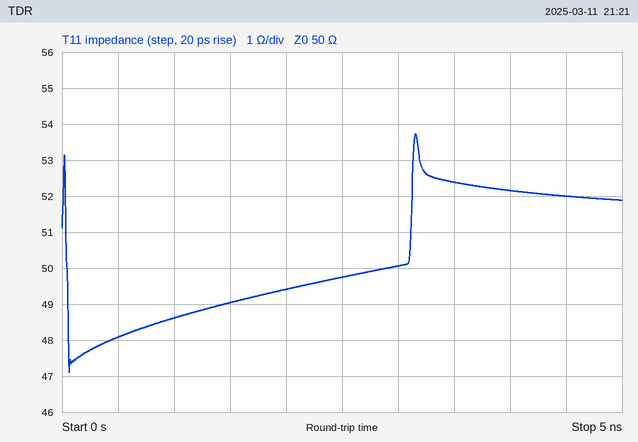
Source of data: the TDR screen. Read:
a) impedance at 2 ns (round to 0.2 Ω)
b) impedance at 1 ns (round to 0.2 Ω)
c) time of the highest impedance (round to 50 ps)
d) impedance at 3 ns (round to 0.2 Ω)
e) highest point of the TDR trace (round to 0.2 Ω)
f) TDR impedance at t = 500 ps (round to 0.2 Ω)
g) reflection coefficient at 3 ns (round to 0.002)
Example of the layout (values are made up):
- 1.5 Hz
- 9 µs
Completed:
- 49.4 Ω
- 48.6 Ω
- 3.15 ns
- 50.0 Ω
- 53.8 Ω
- 48.0 Ω
- 0.000
